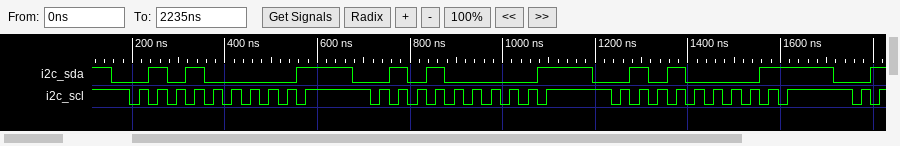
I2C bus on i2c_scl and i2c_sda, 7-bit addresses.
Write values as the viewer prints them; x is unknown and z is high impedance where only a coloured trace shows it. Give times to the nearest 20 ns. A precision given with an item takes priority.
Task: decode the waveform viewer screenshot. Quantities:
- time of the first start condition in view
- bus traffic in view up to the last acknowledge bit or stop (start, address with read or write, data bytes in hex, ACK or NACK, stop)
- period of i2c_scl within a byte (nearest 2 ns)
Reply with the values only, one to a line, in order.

160 ns
start, address 28 write ACK, repeated start, address 28 write ACK, repeated start, address 28 write NACK
40 ns
